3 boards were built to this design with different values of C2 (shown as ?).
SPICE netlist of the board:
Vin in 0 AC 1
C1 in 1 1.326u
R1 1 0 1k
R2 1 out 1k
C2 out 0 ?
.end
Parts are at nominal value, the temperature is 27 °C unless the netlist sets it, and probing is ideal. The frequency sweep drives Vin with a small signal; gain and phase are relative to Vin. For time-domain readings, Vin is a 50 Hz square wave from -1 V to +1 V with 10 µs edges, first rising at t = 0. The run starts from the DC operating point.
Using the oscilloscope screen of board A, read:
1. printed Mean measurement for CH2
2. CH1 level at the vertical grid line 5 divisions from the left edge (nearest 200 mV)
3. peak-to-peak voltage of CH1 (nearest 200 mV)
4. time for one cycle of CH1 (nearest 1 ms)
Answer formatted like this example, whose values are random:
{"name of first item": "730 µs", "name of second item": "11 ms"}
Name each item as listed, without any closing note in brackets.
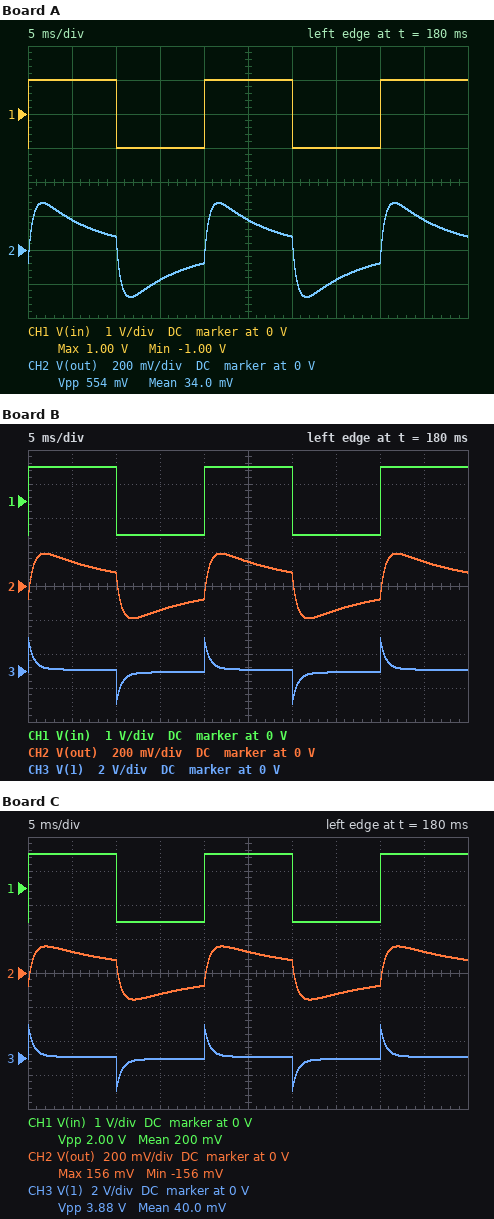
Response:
{"printed Mean measurement for CH2": "34.0 mV", "CH1 level at the vertical grid line 5 divisions from the left edge": "1.0 V", "peak-to-peak voltage of CH1": "2.0 V", "time for one cycle of CH1": "20 ms"}
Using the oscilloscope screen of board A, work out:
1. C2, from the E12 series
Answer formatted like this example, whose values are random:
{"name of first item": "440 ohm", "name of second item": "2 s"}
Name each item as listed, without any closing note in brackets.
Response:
{"C2, from the E12 series": "2.7 µF"}
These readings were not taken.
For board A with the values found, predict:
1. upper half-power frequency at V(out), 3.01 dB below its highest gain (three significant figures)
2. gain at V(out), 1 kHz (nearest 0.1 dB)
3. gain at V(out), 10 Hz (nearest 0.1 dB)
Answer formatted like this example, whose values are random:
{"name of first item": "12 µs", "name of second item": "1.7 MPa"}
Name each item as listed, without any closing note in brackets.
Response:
{"upper half-power frequency at V(out), 3.01 dB below its highest gain": "321 Hz", "gain at V(out), 1 kHz": "-24.9 dB", "gain at V(out), 10 Hz": "-22.2 dB"}
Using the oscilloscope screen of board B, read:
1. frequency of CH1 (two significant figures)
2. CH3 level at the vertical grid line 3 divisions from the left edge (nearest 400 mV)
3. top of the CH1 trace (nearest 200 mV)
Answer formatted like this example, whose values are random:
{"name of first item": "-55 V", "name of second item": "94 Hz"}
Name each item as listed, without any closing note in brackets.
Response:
{"frequency of CH1": "50 Hz", "CH3 level at the vertical grid line 3 divisions from the left edge": "0 V", "top of the CH1 trace": "1.0 V"}
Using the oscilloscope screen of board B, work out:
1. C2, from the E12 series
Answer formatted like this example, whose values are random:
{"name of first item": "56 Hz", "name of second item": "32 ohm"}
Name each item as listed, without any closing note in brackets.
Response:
{"C2, from the E12 series": "3.9 µF"}
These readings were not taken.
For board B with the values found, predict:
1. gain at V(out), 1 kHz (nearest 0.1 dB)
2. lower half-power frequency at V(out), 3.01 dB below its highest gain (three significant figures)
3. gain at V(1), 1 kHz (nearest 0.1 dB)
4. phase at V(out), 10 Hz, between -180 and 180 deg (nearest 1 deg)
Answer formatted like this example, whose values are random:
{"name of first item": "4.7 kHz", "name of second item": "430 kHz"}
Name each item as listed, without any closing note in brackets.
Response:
{"gain at V(out), 1 kHz": "-28.1 dB", "lower half-power frequency at V(out), 3.01 dB below its highest gain": "16.5 Hz", "gain at V(1), 1 kHz": "-0.3 dB", "phase at V(out), 10 Hz, between -180 and 180 deg": "60 deg"}
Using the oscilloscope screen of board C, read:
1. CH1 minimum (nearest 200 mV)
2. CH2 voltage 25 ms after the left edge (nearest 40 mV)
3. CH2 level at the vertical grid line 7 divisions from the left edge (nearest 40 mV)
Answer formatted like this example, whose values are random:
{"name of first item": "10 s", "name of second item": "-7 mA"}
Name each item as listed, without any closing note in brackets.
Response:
{"CH1 minimum": "-1.0 V", "CH2 voltage 25 ms after the left edge": "120 mV", "CH2 level at the vertical grid line 7 divisions from the left edge": "-120 mV"}
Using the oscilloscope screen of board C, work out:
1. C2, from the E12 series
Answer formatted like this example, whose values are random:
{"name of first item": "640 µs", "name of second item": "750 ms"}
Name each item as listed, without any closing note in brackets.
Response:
{"C2, from the E12 series": "4.7 µF"}
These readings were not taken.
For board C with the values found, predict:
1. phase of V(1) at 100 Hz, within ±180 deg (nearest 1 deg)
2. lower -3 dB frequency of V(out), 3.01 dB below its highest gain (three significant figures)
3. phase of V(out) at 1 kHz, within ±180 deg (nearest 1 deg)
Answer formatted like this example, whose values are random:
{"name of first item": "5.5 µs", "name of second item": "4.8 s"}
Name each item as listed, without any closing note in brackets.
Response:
{"phase of V(1) at 100 Hz, within ±180 deg": "59 deg", "lower -3 dB frequency of V(out), 3.01 dB below its highest gain": "14.1 Hz", "phase of V(out) at 1 kHz, within ±180 deg": "-75 deg"}
